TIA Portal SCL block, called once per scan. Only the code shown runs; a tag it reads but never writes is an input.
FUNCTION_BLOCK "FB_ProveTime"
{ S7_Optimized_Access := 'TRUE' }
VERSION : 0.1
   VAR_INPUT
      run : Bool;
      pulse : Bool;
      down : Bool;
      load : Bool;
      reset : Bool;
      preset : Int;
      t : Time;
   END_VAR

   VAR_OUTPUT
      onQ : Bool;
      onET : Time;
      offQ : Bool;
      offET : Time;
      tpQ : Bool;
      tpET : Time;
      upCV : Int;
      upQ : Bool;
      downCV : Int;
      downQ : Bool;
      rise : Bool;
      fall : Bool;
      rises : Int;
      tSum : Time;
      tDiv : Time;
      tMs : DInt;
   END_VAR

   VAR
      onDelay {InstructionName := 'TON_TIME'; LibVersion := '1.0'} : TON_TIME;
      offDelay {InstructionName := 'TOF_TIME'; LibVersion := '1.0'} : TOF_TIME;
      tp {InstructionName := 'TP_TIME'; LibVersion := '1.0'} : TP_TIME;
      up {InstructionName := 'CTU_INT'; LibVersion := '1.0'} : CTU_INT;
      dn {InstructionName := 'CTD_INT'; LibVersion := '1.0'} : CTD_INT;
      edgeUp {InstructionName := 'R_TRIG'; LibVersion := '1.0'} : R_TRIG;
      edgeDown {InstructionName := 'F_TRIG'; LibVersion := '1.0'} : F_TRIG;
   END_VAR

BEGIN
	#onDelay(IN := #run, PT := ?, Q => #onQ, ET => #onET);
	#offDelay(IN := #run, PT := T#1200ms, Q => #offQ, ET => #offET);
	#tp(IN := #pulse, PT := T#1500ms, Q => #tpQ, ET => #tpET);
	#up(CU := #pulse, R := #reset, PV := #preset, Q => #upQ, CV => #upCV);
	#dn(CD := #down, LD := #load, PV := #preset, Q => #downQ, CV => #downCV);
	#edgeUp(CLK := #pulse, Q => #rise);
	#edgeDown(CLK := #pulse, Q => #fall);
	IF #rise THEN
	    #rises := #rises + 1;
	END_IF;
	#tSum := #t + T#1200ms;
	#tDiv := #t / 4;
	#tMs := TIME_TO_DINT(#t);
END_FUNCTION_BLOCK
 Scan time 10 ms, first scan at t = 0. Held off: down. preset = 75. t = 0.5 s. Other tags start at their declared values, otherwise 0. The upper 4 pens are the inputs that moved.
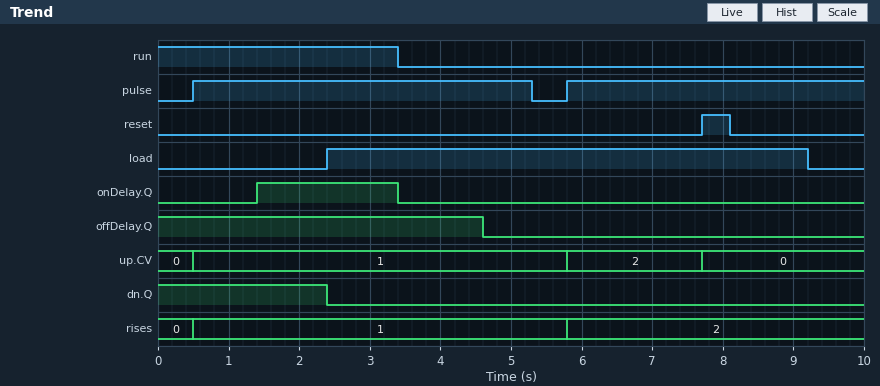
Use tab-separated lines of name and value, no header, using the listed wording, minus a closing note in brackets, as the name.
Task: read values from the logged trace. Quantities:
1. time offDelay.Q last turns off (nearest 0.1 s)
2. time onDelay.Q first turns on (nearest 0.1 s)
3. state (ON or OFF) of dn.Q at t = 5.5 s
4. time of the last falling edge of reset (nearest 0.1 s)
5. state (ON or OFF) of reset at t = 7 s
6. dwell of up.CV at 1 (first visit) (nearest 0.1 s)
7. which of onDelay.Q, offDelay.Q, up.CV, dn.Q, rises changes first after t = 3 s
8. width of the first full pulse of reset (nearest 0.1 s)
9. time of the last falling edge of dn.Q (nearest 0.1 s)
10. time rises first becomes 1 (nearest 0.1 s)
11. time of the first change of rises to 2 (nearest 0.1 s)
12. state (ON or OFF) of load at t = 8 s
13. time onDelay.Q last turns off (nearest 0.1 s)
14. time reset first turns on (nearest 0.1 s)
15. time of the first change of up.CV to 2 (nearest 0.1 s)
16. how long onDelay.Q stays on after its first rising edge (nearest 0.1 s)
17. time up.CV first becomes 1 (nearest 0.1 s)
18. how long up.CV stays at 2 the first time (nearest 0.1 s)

time offDelay.Q last turns off	4.6 s
time onDelay.Q first turns on	1.4 s
state (ON or OFF) of dn.Q at t = 5.5 s	OFF
time of the last falling edge of reset	8.1 s
state (ON or OFF) of reset at t = 7 s	OFF
dwell of up.CV at 1 (first visit)	5.3 s
which of onDelay.Q, offDelay.Q, up.CV, dn.Q, rises changes first after t = 3 s	onDelay.Q
width of the first full pulse of reset	0.4 s
time of the last falling edge of dn.Q	2.4 s
time rises first becomes 1	0.5 s
time of the first change of rises to 2	5.8 s
state (ON or OFF) of load at t = 8 s	ON
time onDelay.Q last turns off	3.4 s
time reset first turns on	7.7 s
time of the first change of up.CV to 2	5.8 s
how long onDelay.Q stays on after its first rising edge	2.0 s
time up.CV first becomes 1	0.5 s
how long up.CV stays at 2 the first time	1.9 s
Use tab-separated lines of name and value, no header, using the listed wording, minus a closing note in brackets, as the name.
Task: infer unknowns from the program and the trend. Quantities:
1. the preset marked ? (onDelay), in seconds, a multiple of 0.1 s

the preset marked ? (onDelay), in seconds, a multiple of 0.1 s	1.4 s
